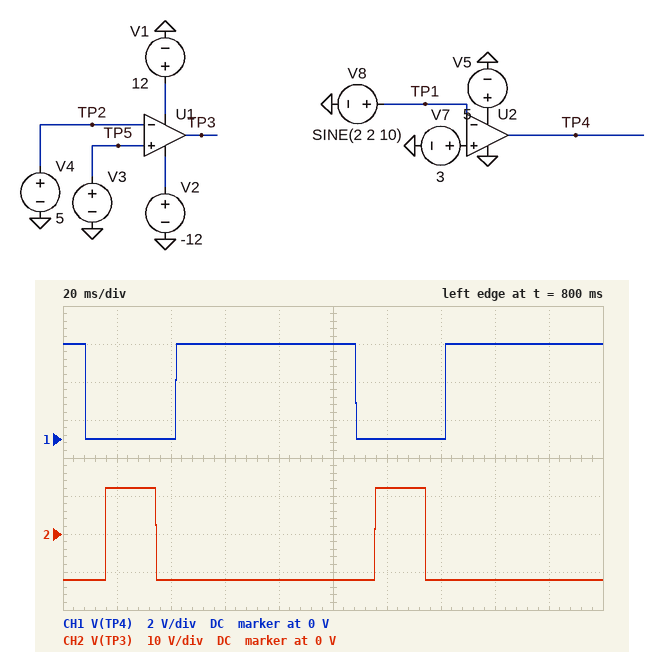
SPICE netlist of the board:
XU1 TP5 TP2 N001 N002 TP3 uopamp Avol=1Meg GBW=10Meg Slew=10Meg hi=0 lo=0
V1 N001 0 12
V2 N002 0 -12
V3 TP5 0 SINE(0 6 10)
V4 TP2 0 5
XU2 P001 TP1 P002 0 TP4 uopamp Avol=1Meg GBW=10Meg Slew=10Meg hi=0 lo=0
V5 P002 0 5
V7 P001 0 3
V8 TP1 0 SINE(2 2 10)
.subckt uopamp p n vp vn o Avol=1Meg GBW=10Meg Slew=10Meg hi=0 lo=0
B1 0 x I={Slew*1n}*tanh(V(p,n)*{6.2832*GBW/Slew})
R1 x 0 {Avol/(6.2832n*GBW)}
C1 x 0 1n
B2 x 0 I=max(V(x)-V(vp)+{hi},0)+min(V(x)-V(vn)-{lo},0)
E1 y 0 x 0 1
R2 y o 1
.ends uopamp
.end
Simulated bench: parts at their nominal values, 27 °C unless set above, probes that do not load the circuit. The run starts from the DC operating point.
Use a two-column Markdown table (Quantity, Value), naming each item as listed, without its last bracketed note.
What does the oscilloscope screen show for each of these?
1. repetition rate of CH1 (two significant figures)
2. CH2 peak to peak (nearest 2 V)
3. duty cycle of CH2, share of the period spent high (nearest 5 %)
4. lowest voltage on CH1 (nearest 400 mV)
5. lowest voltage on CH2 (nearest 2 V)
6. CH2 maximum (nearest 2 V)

| Quantity | Value |
|---|---|
| repetition rate of CH1 | 10 Hz |
| CH2 peak to peak | 24 V |
| duty cycle of CH2, share of the period spent high | 20 % |
| lowest voltage on CH1 | 0 V |
| lowest voltage on CH2 | -12 V |
| CH2 maximum | 12 V |
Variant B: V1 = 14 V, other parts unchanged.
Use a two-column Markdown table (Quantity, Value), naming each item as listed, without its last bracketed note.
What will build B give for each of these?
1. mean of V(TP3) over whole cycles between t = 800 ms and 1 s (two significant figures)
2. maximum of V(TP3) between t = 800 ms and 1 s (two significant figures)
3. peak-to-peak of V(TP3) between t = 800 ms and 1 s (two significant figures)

| Quantity | Value |
|---|---|
| mean of V(TP3) over whole cycles between t = 800 ms and 1 s | -7.2 V |
| maximum of V(TP3) between t = 800 ms and 1 s | 14 V |
| peak-to-peak of V(TP3) between t = 800 ms and 1 s | 26 V |
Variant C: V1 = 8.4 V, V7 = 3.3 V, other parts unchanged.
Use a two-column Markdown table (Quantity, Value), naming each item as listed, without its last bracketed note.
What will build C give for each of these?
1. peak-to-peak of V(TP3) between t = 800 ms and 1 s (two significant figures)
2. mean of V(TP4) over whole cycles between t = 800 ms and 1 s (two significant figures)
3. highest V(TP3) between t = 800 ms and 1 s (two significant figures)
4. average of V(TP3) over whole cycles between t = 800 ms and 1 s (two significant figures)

| Quantity | Value |
|---|---|
| peak-to-peak of V(TP3) between t = 800 ms and 1 s | 20 V |
| mean of V(TP4) over whole cycles between t = 800 ms and 1 s | 3.6 V |
| highest V(TP3) between t = 800 ms and 1 s | 8.4 V |
| average of V(TP3) over whole cycles between t = 800 ms and 1 s | -8.2 V |
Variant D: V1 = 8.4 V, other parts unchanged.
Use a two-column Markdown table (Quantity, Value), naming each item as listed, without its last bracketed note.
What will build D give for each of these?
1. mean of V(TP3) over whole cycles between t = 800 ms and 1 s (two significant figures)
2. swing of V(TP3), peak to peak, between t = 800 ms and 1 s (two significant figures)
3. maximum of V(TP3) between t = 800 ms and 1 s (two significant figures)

| Quantity | Value |
|---|---|
| mean of V(TP3) over whole cycles between t = 800 ms and 1 s | -8.2 V |
| swing of V(TP3), peak to peak, between t = 800 ms and 1 s | 20 V |
| maximum of V(TP3) between t = 800 ms and 1 s | 8.4 V |
